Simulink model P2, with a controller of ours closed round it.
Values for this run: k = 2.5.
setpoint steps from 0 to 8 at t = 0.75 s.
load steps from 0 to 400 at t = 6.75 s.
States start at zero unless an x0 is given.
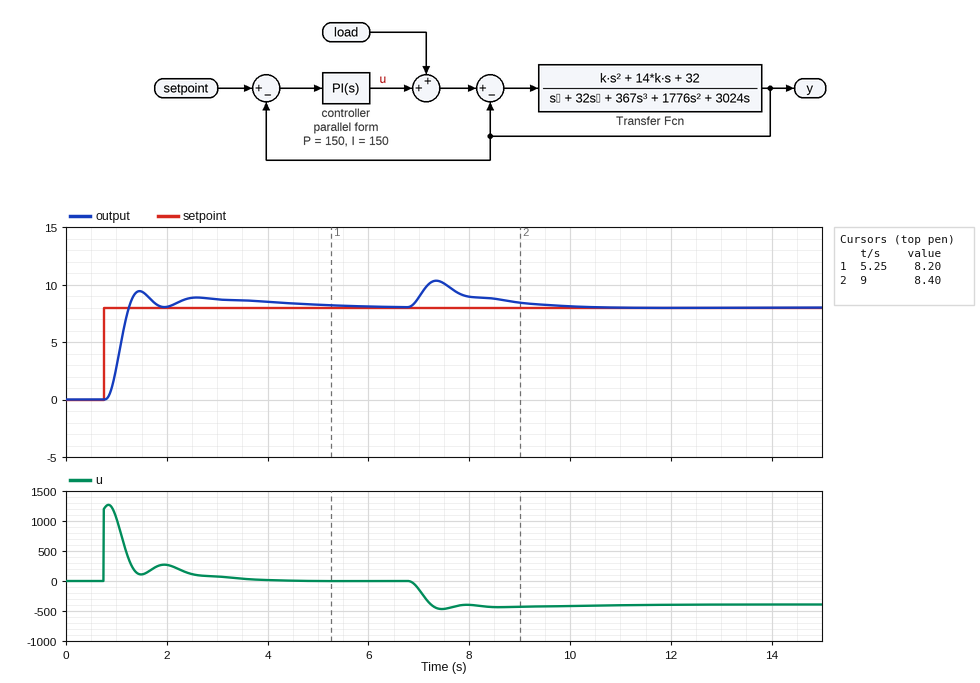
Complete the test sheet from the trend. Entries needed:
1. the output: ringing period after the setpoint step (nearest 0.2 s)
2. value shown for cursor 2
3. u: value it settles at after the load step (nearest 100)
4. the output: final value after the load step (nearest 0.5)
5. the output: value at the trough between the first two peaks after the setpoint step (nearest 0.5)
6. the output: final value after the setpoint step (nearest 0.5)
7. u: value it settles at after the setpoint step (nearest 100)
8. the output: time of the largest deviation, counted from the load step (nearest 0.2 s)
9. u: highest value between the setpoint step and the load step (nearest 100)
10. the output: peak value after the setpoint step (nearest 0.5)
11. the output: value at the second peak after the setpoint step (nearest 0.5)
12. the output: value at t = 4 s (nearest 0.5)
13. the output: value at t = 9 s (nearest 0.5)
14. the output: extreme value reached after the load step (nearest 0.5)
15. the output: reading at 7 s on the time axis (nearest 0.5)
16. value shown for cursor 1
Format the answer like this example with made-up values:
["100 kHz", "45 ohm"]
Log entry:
["1.2 s", "8.40", "-400", "8.0", "8.0", "8.0", "0", "0.6 s", "1300", "9.5", "9.0", "8.5", "8.5", "10.5", "9.0", "8.20"]
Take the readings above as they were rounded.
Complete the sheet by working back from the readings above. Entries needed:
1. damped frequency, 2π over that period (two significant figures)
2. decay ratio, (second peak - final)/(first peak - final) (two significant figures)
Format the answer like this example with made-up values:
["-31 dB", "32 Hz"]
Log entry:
["5.2 rad/s", "0.67"]
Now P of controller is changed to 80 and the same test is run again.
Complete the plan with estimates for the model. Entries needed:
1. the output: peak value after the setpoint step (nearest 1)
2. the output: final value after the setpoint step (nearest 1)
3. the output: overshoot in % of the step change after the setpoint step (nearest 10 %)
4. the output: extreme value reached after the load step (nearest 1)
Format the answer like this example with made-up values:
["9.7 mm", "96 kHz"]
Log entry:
["10", "8", "20 %", "11"]
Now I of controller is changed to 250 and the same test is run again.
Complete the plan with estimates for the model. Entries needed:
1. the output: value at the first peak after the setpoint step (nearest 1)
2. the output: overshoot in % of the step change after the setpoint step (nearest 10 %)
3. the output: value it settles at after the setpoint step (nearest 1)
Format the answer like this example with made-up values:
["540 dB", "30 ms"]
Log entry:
["11", "30 %", "8"]
